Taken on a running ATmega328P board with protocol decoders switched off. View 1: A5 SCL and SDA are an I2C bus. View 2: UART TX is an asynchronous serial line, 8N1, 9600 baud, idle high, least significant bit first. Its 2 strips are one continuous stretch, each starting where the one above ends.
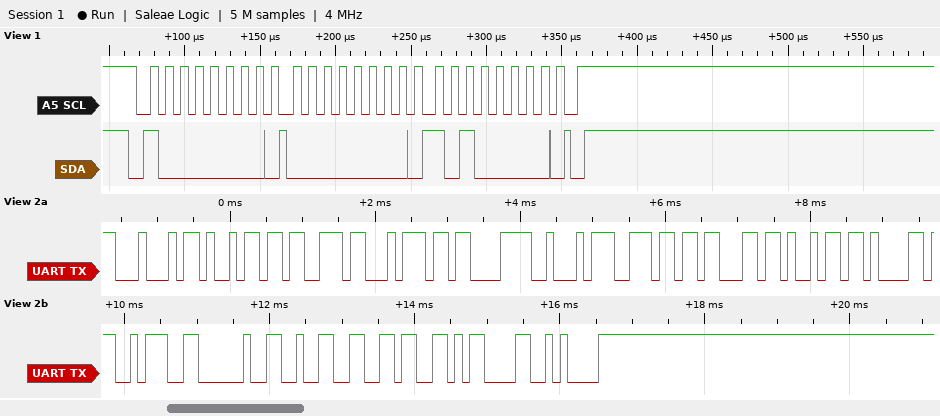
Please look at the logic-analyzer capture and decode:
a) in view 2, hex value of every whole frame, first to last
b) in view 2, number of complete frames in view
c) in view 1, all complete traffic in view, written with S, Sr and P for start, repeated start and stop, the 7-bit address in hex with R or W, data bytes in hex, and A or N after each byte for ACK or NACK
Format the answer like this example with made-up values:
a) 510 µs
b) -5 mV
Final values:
a) 0x44 0x69 0x73 0x74 0xC3 0xA2 0x6E 0x63 0x69 0x61 0x3A 0x20 0x32 0x36 0x0D 0x0A
b) 16
c) S 40W A 00 A A0 A P
